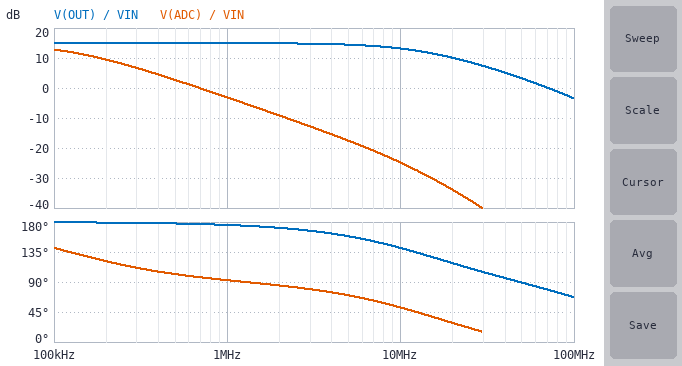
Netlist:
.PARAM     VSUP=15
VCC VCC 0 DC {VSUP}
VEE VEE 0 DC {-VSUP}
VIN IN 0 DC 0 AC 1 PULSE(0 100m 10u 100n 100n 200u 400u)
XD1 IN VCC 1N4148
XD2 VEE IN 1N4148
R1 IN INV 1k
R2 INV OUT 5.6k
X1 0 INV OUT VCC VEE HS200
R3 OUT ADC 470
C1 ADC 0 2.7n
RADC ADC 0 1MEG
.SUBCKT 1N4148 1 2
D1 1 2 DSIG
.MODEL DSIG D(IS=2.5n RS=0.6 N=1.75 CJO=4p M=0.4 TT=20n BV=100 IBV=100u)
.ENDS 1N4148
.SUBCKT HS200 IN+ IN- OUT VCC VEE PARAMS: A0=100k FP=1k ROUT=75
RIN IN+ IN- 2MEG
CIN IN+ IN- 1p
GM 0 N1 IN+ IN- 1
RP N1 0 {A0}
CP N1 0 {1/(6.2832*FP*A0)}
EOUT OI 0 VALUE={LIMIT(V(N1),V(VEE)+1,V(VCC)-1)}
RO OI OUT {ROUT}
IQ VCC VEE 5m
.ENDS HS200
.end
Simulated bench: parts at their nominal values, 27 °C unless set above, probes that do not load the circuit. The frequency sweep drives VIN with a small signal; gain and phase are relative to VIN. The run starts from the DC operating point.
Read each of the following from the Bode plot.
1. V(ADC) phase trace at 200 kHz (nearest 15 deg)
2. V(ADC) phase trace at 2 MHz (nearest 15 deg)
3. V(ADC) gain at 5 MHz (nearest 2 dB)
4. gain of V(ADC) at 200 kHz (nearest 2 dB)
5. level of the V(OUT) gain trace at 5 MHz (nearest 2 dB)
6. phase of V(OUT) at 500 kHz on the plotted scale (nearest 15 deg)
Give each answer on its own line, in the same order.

120 deg
90 deg
-18 dB
10 dB
14 dB
180 deg
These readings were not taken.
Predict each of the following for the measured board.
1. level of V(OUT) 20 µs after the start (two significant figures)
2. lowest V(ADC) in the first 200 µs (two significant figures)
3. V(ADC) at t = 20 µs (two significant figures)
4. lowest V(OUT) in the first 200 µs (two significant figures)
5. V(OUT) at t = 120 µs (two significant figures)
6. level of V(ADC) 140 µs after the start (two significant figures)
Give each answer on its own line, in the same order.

-560 mV
-560 mV
-560 mV
-560 mV
-560 mV
-560 mV
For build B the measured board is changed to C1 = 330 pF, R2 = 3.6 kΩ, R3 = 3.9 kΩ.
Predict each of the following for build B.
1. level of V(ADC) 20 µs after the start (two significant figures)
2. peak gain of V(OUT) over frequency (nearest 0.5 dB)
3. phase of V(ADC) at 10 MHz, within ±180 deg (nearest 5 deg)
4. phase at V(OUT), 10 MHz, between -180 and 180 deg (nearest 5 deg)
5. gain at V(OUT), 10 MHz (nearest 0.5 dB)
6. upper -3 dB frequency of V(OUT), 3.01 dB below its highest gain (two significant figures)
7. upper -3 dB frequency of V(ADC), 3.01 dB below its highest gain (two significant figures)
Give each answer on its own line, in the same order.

-360 mV
11.0 dB
65 deg
155 deg
10.5 dB
23 MHz
120 kHz
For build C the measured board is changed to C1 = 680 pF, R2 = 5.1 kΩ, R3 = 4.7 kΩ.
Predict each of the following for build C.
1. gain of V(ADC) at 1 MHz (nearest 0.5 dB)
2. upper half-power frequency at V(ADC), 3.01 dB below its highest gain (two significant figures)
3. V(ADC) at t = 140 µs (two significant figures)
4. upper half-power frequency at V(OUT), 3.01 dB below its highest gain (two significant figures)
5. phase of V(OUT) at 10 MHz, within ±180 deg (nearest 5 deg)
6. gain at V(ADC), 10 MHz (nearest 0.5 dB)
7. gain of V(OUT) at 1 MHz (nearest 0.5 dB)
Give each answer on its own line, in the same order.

-12.0 dB
50 kHz
-510 mV
17 MHz
145 deg
-33.0 dB
14.0 dB
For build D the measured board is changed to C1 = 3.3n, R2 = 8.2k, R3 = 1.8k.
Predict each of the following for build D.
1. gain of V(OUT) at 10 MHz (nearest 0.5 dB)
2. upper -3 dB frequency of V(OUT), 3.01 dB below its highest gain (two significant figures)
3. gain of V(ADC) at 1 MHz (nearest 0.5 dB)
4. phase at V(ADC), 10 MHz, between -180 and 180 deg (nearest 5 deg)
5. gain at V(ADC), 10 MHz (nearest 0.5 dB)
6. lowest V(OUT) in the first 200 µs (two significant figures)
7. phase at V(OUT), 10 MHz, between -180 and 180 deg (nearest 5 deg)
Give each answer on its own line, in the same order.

15.5 dB
11 MHz
-13.0 dB
45 deg
-36.0 dB
-820 mV
135 deg
